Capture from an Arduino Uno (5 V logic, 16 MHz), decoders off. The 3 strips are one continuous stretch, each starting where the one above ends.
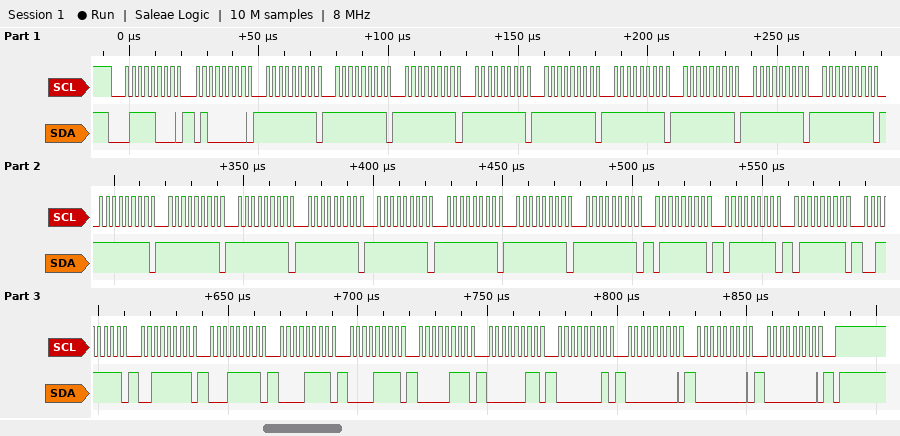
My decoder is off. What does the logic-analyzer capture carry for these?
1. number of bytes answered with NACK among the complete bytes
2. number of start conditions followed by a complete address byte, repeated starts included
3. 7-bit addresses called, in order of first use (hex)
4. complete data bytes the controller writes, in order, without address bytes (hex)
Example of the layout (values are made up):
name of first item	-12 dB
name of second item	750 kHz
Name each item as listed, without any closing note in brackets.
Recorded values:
number of bytes answered with NACK among the complete bytes	0
number of start conditions followed by a complete address byte, repeated starts included	1
7-bit addresses called, in order of first use	0x3C
complete data bytes the controller writes, in order, without address bytes	40 FF FF FF FF FF FF FF FF FF FF FF FF FF FF FF FF FF 7F 7F 7F 3F 3F 1F 0F 0F 07 03 01 00 00 00
